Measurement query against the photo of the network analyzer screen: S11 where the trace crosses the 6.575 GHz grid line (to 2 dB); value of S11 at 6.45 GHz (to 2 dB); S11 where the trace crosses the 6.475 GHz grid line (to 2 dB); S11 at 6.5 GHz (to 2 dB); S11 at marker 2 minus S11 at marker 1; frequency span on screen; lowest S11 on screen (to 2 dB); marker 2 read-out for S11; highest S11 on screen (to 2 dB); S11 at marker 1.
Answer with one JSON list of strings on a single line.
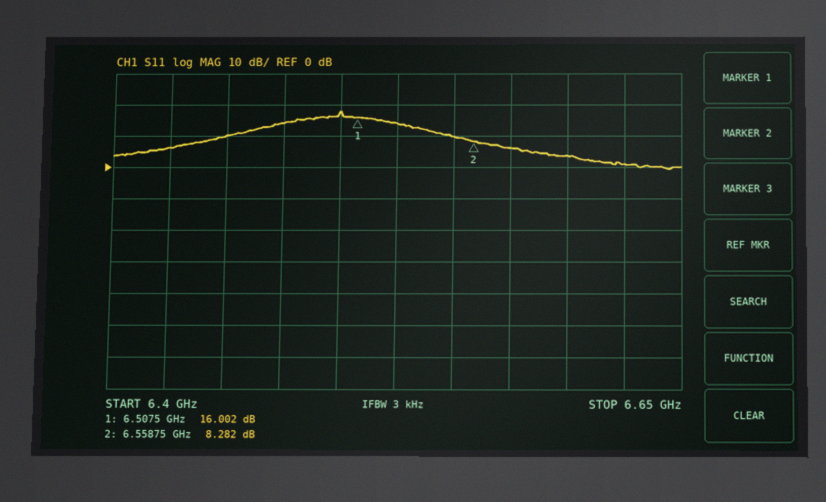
["6 dB", "10 dB", "14 dB", "18 dB", "-7.720 dB", "250 MHz", "0 dB", "8.282 dB", "18 dB", "16.002 dB"]
